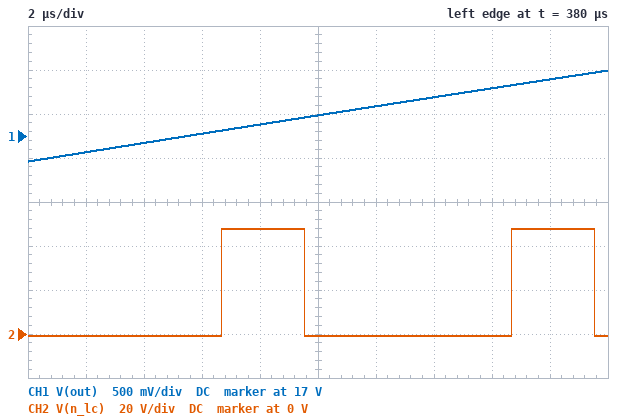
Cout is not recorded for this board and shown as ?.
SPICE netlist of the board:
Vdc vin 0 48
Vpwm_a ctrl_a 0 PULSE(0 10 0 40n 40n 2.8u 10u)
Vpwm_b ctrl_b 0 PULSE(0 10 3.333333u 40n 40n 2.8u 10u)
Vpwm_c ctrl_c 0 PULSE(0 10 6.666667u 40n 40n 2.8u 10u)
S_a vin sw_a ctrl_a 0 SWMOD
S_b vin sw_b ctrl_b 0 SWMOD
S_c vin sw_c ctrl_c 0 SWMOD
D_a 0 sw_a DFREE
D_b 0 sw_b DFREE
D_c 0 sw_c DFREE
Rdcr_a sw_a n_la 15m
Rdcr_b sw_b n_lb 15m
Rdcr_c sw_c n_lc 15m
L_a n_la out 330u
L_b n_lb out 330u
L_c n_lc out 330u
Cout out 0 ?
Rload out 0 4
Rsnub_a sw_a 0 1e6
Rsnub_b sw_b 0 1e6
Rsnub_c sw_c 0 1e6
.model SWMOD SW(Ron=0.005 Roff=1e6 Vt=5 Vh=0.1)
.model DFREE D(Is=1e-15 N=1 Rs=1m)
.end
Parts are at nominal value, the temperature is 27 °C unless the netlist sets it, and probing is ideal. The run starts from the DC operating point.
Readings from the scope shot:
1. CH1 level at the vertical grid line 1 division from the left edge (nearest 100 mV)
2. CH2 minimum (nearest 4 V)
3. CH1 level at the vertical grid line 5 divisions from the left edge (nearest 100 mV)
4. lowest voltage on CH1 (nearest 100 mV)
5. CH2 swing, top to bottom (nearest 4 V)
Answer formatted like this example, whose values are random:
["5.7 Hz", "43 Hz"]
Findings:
["16.8 V", "0 V", "17.2 V", "16.7 V", "48 V"]
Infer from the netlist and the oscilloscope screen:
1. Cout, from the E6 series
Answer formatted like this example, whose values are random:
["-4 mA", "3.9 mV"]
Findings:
["330 µF"]
